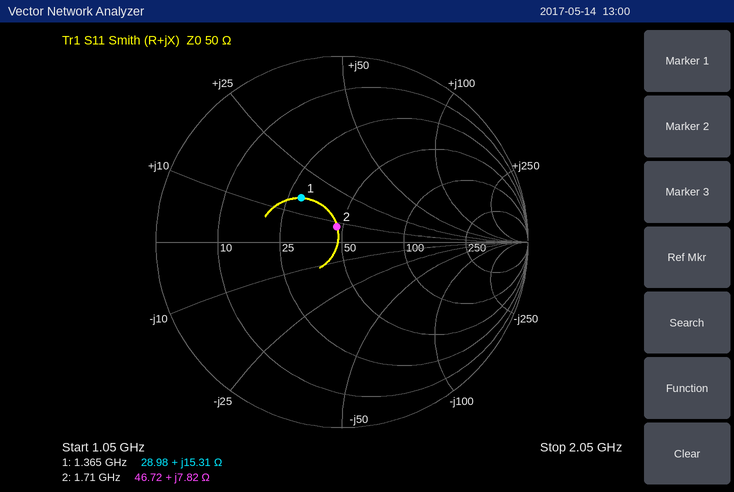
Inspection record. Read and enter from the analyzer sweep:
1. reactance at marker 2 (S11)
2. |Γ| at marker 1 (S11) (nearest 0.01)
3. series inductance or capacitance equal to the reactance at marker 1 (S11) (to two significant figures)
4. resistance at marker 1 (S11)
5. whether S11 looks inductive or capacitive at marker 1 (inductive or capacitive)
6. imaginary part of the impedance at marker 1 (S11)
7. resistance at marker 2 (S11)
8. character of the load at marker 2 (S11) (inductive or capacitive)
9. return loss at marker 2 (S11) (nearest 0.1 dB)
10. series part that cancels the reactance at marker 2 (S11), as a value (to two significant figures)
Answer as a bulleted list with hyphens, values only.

- +7.82 Ω
- 0.32
- 1.8 nH
- 28.98 Ω
- inductive
- +15.31 Ω
- 46.72 Ω
- inductive
- 21.2 dB
- 12 pF
